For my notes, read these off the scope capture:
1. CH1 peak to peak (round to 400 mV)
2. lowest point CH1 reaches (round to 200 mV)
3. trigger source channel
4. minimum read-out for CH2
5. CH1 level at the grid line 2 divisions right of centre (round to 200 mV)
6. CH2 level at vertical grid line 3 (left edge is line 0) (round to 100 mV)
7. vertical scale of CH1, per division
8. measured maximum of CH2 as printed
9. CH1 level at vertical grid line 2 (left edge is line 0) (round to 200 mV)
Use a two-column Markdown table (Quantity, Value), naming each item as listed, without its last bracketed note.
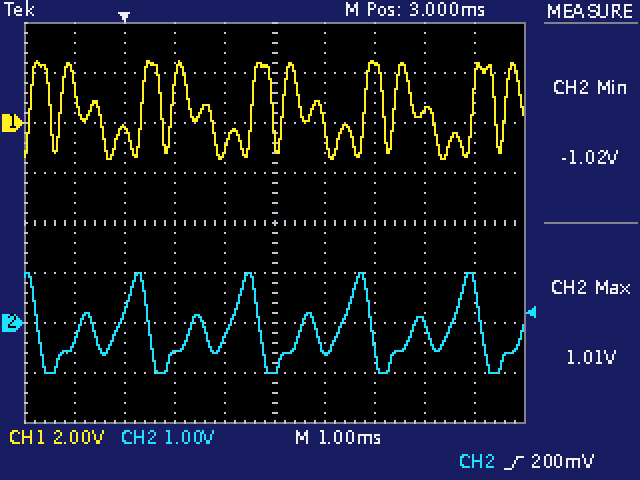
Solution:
| Quantity | Value |
|---|---|
| CH1 peak to peak | 4.0 V |
| lowest point CH1 reaches | -1.4 V |
| trigger source channel | CH2 |
| minimum read-out for CH2 | -1.02 V |
| CH1 level at the grid line 2 divisions right of centre | 2.4 V |
| CH2 level at vertical grid line 3 (left edge is line 0) | -600 mV |
| vertical scale of CH1, per division | 2 V |
| measured maximum of CH2 as printed | 1.01 V |
| CH1 level at vertical grid line 2 (left edge is line 0) | -200 mV |
